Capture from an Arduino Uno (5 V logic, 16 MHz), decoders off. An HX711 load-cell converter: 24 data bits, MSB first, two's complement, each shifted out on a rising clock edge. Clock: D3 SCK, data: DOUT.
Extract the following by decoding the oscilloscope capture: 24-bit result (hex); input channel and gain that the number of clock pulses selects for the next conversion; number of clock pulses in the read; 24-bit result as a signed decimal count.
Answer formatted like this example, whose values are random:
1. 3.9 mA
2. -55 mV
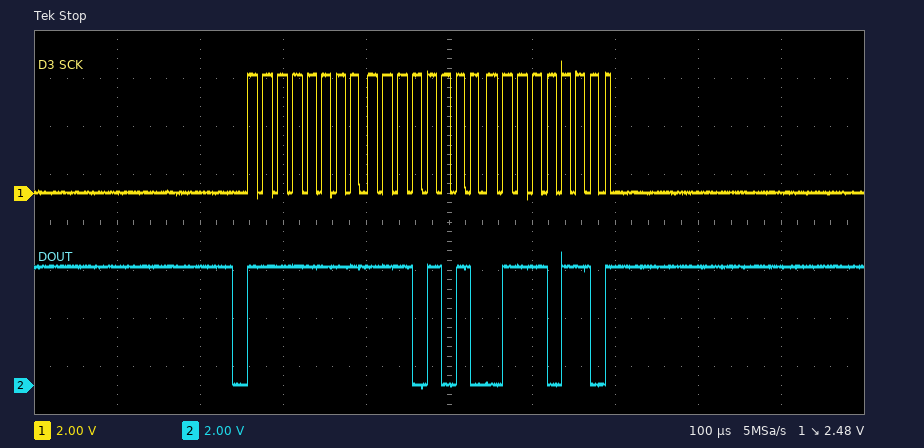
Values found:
1. 0xFFEA76
2. channel A, gain 128
3. 25
4. -5514
